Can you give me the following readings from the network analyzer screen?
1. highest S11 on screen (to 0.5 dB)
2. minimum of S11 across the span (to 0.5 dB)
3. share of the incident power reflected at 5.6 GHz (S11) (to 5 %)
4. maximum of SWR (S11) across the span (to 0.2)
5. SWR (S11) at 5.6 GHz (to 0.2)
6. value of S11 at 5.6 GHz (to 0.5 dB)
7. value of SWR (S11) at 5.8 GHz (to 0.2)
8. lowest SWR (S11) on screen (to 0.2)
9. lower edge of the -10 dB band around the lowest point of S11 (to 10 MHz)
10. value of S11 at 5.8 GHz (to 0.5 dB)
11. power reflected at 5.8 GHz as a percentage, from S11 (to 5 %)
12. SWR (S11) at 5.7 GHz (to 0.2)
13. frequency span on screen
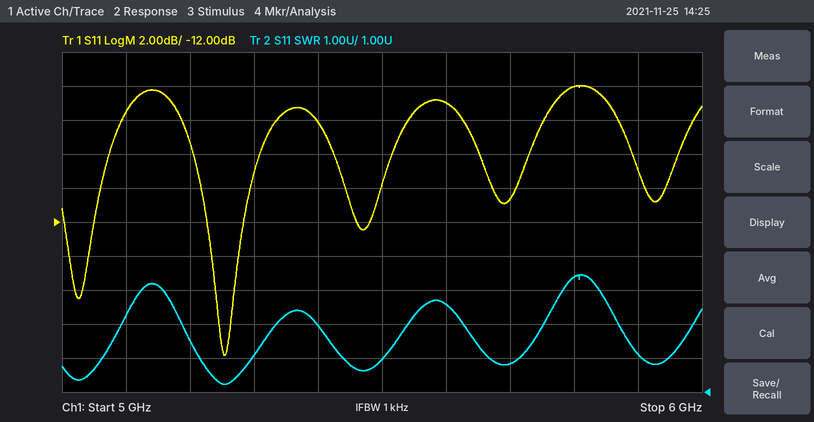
-4.0 dB
-20.0 dB
30 %
4.4
3.6
-5.0 dB
4.4
1.2
5.22 GHz
-4.0 dB
40 %
1.8
1 GHz
